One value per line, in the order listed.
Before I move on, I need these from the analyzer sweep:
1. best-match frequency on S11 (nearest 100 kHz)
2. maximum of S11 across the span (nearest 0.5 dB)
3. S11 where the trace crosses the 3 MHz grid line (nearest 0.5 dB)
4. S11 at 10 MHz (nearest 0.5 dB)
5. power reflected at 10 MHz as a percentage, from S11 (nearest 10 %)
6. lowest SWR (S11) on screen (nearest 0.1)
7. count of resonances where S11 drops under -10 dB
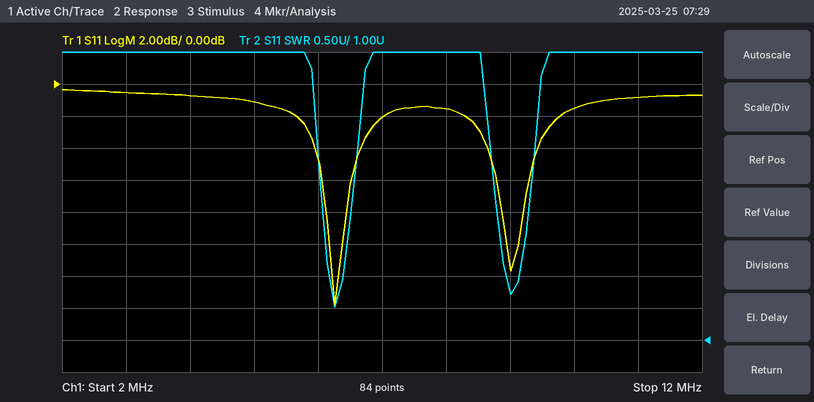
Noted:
6.3 MHz
-0.5 dB
-0.5 dB
-1.5 dB
70 %
1.5
2
